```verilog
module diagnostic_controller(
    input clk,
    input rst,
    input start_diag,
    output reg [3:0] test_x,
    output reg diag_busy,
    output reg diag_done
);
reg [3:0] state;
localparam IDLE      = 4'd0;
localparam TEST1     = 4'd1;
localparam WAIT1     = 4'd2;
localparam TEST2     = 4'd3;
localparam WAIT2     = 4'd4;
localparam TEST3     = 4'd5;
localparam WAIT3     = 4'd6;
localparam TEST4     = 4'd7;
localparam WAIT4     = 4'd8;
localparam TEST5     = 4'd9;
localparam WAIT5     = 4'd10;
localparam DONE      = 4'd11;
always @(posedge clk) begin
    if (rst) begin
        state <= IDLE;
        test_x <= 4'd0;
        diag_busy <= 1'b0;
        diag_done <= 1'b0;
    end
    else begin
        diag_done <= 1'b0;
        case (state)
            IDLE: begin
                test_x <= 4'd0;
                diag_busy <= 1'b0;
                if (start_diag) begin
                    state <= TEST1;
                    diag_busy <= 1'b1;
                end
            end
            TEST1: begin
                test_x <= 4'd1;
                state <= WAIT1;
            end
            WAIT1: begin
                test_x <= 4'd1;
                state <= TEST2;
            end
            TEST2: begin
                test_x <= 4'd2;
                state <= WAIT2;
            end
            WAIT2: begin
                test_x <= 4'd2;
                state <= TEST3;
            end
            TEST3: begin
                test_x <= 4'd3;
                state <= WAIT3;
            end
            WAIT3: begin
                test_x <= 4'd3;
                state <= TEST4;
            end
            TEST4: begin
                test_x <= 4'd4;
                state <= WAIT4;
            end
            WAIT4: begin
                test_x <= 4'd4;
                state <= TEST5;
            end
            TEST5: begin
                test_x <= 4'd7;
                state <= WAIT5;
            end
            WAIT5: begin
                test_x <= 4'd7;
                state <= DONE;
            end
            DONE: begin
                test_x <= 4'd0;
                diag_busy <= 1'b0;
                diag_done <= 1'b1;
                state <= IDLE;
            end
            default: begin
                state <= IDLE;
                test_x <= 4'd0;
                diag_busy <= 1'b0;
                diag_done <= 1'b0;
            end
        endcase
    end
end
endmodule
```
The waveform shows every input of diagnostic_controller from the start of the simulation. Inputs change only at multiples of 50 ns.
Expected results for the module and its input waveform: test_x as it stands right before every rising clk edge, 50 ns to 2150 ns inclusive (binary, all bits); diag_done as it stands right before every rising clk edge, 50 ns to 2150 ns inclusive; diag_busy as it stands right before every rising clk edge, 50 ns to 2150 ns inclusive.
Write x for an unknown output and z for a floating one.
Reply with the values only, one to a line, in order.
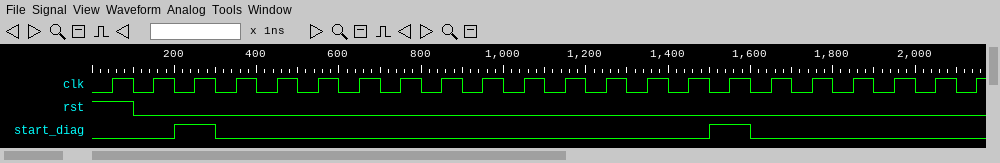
x, 0000, 0000, 0000, 0001, 0001, 0010, 0010, 0011, 0011, 0100, 0100, 0111, 0111, 0000, 0000, 0000, 0001, 0001, 0010, 0010, 0011
x 0 0 0 0 0 0 0 0 0 0 0 0 0 1 0 0 0 0 0 0 0
x 0 0 1 1 1 1 1 1 1 1 1 1 1 0 0 1 1 1 1 1 1
